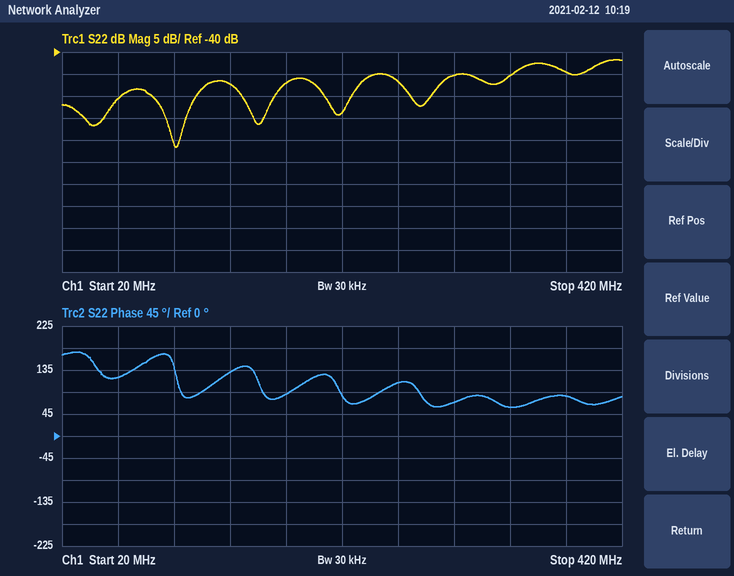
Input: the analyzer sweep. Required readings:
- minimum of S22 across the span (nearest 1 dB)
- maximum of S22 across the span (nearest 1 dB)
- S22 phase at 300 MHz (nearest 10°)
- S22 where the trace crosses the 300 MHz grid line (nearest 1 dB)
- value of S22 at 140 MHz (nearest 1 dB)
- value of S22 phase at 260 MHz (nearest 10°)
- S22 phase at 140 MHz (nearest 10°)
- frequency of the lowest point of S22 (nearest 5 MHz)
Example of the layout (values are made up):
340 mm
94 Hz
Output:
-62 dB
-42 dB
70°
-45 dB
-47 dB
110°
130°
100 MHz
